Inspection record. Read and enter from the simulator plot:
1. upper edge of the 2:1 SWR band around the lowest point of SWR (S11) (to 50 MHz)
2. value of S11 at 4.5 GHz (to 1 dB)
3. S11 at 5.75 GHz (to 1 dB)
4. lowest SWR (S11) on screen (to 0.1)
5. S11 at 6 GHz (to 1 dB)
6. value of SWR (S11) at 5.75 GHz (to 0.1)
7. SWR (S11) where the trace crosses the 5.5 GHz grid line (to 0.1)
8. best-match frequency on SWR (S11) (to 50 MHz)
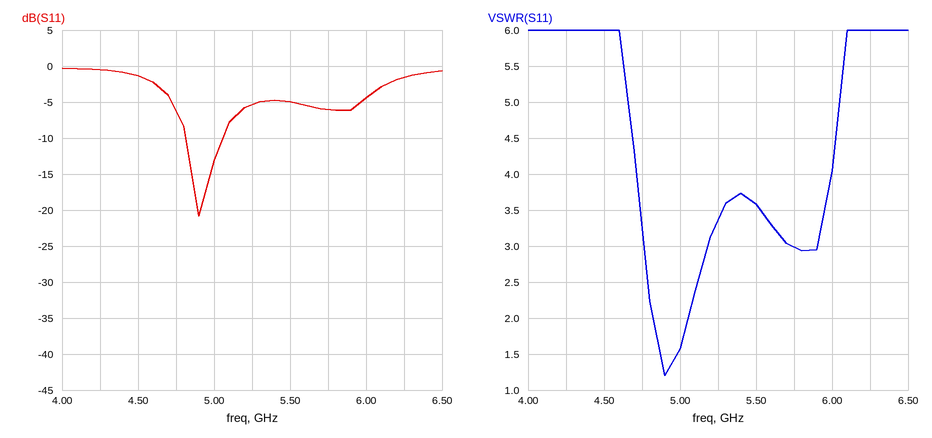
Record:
5.05 GHz
-1 dB
-6 dB
1.2
-4 dB
3.0
3.6
4.90 GHz
